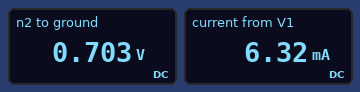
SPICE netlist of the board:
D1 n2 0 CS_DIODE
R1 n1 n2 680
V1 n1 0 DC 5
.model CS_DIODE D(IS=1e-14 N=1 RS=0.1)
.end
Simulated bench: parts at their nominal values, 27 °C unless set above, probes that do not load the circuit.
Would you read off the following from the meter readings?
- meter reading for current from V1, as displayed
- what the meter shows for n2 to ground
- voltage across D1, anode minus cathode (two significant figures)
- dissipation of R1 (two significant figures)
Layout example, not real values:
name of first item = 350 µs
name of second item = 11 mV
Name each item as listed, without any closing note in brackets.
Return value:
meter reading for current from V1, as displayed = 6.32 mA
what the meter shows for n2 to ground = 0.703 V
voltage across D1, anode minus cathode = 700 mV
dissipation of R1 = 27 mW
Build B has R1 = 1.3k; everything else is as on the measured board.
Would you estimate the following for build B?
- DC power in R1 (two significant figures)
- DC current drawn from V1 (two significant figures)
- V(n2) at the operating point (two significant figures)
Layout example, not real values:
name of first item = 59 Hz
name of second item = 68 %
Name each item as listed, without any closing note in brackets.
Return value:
DC power in R1 = 14 mW
DC current drawn from V1 = 3.3 mA
V(n2) at the operating point = 690 mV
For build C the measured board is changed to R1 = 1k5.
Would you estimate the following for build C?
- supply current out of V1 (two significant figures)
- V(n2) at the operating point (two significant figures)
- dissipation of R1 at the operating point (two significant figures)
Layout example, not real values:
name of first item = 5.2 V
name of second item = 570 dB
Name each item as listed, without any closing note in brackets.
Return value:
supply current out of V1 = 2.9 mA
V(n2) at the operating point = 680 mV
dissipation of R1 at the operating point = 12 mW
